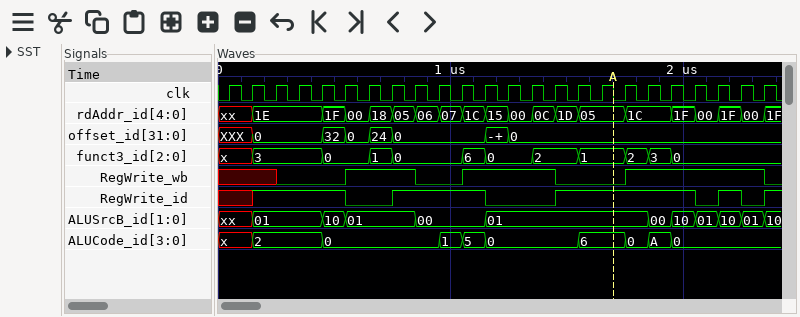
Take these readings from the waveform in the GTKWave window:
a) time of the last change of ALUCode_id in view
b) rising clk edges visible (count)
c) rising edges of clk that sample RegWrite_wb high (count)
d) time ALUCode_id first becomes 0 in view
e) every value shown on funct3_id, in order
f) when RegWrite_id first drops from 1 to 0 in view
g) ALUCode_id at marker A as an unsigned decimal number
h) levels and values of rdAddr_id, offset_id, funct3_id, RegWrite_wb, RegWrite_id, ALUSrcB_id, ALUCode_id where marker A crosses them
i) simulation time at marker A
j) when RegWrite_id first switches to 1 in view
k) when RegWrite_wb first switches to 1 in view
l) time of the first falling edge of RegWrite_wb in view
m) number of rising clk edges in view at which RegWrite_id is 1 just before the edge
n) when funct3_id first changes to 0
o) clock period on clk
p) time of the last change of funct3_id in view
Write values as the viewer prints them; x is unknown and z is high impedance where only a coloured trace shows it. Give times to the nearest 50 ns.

1950 ns
24
13
450 ns
x, 3, 0, 1, 0, 6, 0, 2, 1, 2, 3, 0
550 ns
6
rdAddr_id=05, offset_id=0, funct3_id=1, RegWrite_wb=0, RegWrite_id=1, ALUSrcB_id=01, ALUCode_id=6
1700 ns
150 ns
550 ns
850 ns
15
450 ns
100 ns
1950 ns
